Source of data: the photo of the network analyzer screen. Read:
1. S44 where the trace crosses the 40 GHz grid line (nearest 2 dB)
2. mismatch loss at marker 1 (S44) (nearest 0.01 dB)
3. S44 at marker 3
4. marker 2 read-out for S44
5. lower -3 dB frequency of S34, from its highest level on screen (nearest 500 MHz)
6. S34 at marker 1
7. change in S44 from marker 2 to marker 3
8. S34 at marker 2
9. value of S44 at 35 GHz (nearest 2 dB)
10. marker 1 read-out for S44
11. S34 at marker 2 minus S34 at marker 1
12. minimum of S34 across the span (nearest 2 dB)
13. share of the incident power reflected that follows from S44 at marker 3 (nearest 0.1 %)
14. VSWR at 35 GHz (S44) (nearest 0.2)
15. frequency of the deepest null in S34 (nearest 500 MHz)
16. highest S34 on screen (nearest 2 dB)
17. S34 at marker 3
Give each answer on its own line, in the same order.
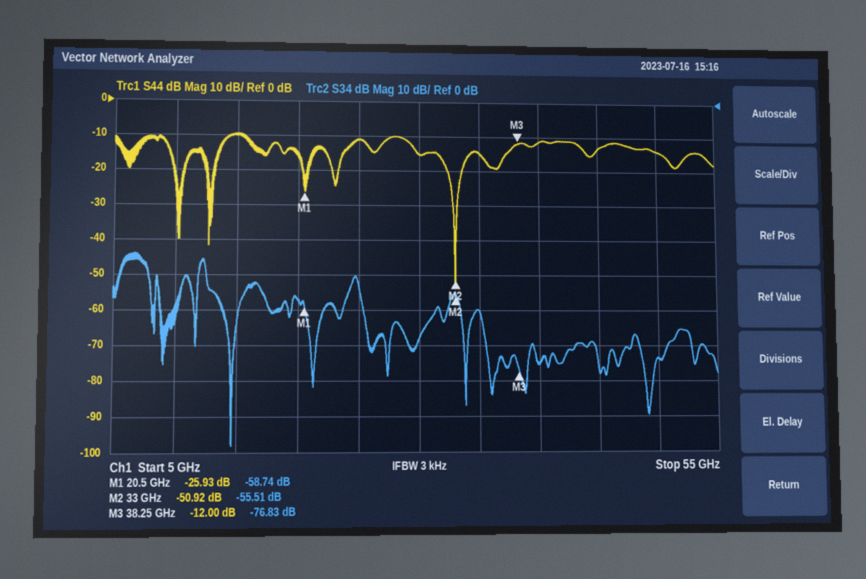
-12 dB
0.01 dB
-12.00 dB
-50.92 dB
6.0 GHz
-58.74 dB
38.92 dB
-55.51 dB
-14 dB
-25.93 dB
3.23 dB
-98 dB
6.3 %
1.4
14.5 GHz
-44 dB
-76.83 dB
